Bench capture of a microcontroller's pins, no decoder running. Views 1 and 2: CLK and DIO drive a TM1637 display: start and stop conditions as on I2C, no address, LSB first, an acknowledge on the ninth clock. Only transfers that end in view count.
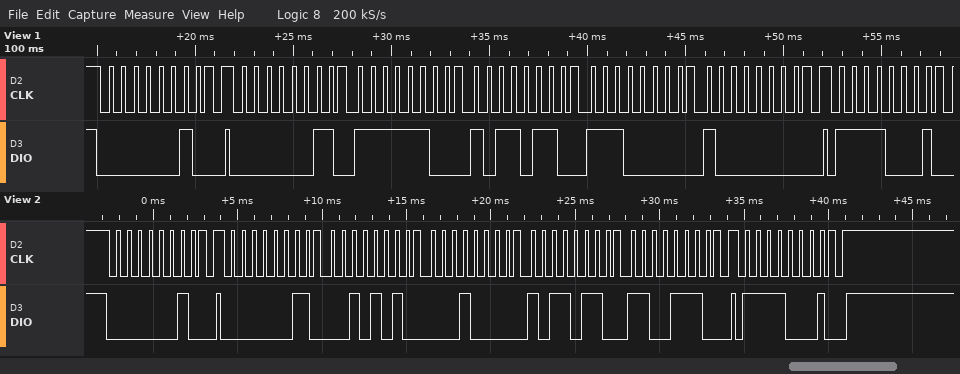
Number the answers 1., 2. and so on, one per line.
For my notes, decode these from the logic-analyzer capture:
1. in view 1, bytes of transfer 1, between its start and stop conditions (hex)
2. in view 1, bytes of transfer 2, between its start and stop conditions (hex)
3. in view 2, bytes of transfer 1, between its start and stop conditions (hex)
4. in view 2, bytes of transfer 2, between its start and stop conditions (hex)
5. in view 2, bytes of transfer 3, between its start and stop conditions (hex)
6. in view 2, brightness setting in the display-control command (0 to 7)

1. 40
2. C0 3F 6D 07 01
3. 40
4. C0 54 08 6D 73
5. 8F
6. 7
